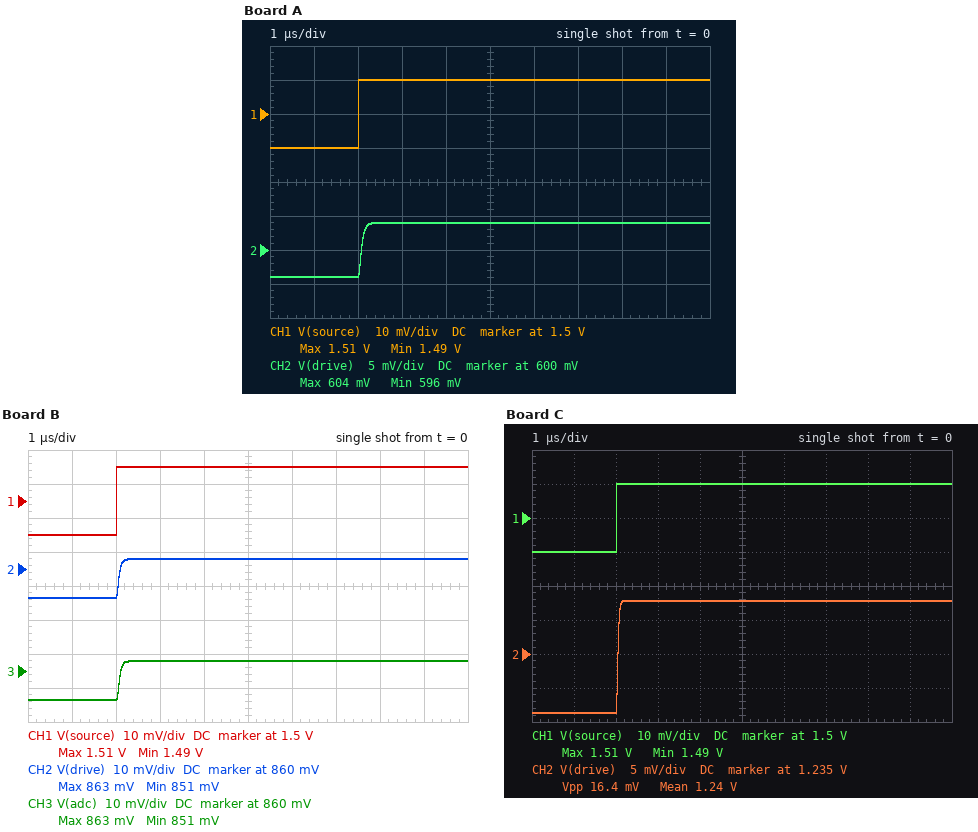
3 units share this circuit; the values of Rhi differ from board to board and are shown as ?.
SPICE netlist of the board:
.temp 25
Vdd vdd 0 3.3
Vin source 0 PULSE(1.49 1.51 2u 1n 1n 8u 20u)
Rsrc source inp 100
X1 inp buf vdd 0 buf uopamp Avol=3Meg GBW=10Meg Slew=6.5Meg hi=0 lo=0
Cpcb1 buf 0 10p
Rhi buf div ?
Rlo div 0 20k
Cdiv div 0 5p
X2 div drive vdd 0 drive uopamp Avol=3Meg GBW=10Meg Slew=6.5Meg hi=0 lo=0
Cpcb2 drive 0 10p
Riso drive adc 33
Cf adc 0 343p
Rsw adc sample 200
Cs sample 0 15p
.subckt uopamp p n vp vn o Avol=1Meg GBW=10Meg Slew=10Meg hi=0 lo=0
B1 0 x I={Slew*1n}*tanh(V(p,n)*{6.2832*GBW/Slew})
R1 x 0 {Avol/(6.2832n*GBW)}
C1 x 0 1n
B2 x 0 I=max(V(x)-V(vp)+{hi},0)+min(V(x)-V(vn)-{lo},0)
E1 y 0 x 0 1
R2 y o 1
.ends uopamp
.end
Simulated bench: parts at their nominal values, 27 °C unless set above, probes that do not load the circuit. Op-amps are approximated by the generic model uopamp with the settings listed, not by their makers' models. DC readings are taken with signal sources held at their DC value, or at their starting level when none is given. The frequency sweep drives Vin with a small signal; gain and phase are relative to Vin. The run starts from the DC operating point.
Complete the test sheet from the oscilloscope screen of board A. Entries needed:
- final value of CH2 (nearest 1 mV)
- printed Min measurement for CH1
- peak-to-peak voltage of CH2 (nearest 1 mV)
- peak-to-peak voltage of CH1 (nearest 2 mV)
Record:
604 mV
1.49 V
8 mV
20 mV
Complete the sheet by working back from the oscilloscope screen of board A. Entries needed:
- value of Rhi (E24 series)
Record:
30 kΩ
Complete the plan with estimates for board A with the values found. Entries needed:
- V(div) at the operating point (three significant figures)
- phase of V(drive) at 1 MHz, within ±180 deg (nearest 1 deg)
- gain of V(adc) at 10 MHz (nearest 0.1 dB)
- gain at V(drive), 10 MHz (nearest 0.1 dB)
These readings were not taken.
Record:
596 mV
-32 deg
-27.7 dB
-25.8 dB
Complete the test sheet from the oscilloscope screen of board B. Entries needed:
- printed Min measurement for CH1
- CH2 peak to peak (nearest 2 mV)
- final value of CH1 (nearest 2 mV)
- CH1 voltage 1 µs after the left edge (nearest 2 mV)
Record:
1.49 V
12 mV
1.510 V
1.490 V
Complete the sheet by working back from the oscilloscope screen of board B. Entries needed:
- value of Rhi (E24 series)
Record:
15 kΩ
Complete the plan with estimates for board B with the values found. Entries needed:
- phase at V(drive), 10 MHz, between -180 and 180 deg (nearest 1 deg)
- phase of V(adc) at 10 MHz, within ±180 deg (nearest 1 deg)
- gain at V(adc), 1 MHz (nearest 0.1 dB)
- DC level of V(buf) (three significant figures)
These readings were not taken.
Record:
-160 deg
163 deg
-5.3 dB
1.49 V
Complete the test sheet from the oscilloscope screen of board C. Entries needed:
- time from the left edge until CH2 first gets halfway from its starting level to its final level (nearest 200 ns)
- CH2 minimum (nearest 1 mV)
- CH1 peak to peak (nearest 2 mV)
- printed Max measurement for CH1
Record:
2.0 µs
1.226 V
20 mV
1.51 V
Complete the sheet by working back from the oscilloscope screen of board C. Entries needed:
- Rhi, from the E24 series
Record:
4.3 kΩ
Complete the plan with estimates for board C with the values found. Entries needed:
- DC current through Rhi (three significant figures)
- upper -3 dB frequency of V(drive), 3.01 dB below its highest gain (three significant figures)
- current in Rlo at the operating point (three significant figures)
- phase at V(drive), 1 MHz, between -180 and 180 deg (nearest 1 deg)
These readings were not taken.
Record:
61.3 µA
4.94 MHz
61.3 µA
-18 deg
